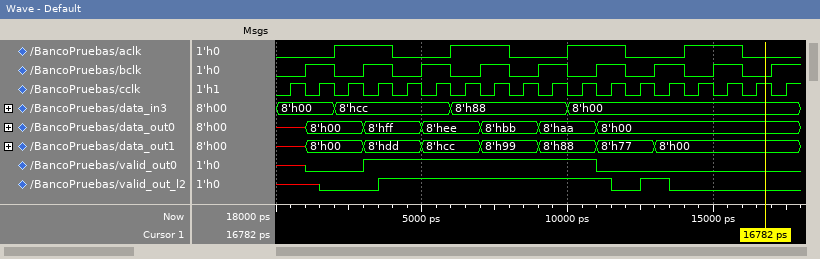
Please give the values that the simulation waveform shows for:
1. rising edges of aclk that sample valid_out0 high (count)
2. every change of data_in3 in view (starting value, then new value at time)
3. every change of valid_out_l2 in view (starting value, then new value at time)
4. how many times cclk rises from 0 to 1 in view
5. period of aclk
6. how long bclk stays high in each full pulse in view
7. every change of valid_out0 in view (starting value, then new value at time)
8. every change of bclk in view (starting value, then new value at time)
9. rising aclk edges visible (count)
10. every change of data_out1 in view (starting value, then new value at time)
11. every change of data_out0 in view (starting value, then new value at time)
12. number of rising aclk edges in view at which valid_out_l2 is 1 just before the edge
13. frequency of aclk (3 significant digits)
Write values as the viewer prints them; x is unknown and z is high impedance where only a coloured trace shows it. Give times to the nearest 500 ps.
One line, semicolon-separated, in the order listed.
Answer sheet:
2; 8'h00, 8'hcc at 2000 ps, 8'h88 at 6000 ps, 8'h00 at 10000 ps; x, 0 at 1500 ps, 1 at 3500 ps, 0 at 11500 ps, 1 at 12500 ps, 0 at 13500 ps; 18; 4000 ps; 1000 ps, 1000 ps, 1000 ps, 1000 ps, 1000 ps, 1000 ps, 1000 ps, 1000 ps; x, 0 at 1000 ps, 1 at 3000 ps, 0 at 11000 ps; 0, 1 at 1000 ps, 0 at 2000 ps, 1 at 3000 ps, 0 at 4000 ps, 1 at 5000 ps, 0 at 6000 ps, 1 at 7000 ps, 0 at 8000 ps, 1 at 9000 ps, 0 at 10000 ps, 1 at 11000 ps, 0 at 12000 ps, 1 at 13000 ps, 0 at 14000 ps, 1 at 15000 ps, 0 at 16000 ps, 1 at 17000 ps; 4; x, 8'h00 at 1000 ps, 8'hdd at 3000 ps, 8'hcc at 5000 ps, 8'h99 at 7000 ps, 8'h88 at 9000 ps, 8'h77 at 11000 ps, 8'h00 at 13000 ps; x, 8'h00 at 1000 ps, 8'hff at 3000 ps, 8'hee at 5000 ps, 8'hbb at 7000 ps, 8'haa at 9000 ps, 8'h00 at 11000 ps; 2; 250 MHz
